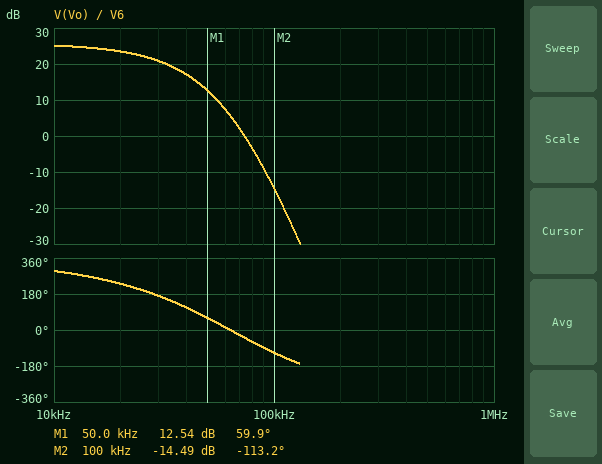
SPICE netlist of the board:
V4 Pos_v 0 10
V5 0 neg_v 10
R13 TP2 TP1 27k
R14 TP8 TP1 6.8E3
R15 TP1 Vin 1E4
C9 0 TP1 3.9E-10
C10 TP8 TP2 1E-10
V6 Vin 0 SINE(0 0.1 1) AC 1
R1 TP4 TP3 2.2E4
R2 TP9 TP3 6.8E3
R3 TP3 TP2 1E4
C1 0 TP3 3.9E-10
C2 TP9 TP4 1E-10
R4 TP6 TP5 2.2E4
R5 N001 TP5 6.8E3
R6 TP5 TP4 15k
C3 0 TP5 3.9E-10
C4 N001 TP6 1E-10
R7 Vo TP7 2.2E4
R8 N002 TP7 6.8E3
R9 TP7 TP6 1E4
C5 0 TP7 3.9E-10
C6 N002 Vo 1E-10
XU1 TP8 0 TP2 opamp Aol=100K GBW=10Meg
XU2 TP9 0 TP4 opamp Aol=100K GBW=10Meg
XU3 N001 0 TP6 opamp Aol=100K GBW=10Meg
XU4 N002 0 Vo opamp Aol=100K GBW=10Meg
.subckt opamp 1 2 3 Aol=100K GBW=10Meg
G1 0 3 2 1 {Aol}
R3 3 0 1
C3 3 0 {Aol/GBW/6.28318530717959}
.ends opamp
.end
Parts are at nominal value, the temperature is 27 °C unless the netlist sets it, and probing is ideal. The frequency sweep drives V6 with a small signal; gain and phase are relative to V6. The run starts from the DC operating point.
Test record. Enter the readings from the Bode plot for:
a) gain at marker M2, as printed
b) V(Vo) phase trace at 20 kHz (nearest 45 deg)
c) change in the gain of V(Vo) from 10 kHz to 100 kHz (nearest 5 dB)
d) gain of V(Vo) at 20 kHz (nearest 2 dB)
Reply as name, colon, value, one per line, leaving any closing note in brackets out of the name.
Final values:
gain at marker M2, as printed: -14.49 dB
V(Vo) phase trace at 20 kHz: 225 deg
change in the gain of V(Vo) from 10 kHz to 100 kHz: -40 dB
gain of V(Vo) at 20 kHz: 24 dB
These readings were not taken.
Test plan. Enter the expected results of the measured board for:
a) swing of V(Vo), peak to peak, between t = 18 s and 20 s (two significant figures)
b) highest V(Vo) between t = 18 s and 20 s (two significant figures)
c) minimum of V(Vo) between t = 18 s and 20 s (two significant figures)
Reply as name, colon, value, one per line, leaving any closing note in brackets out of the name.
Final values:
swing of V(Vo), peak to peak, between t = 18 s and 20 s: 3.8 V
highest V(Vo) between t = 18 s and 20 s: 1.9 V
minimum of V(Vo) between t = 18 s and 20 s: -1.9 V
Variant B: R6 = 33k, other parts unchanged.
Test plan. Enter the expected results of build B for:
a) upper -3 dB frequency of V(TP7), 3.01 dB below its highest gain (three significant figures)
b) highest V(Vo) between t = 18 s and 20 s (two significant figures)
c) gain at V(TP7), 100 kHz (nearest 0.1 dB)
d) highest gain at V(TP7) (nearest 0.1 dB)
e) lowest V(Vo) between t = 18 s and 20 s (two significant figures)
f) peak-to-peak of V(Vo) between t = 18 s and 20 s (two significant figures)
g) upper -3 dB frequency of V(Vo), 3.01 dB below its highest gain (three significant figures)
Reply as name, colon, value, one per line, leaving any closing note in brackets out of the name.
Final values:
upper -3 dB frequency of V(TP7), 3.01 dB below its highest gain: 49.3 kHz
highest V(Vo) between t = 18 s and 20 s: 870 mV
gain at V(TP7), 100 kHz: -27.5 dB
highest gain at V(TP7): -3.1 dB
lowest V(Vo) between t = 18 s and 20 s: -870 mV
peak-to-peak of V(Vo) between t = 18 s and 20 s: 1.7 V
upper -3 dB frequency of V(Vo), 3.01 dB below its highest gain: 25.2 kHz
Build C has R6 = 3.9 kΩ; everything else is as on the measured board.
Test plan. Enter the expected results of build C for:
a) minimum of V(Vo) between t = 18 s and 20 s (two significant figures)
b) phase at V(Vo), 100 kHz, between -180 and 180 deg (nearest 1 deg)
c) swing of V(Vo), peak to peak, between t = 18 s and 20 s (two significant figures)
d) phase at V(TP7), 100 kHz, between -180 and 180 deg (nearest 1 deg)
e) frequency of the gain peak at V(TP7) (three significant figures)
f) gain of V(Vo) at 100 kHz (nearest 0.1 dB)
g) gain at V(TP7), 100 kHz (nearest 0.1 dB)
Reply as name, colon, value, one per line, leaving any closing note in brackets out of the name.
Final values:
minimum of V(Vo) between t = 18 s and 20 s: -7.4 V
phase at V(Vo), 100 kHz, between -180 and 180 deg: -102 deg
swing of V(Vo), peak to peak, between t = 18 s and 20 s: 15 V
phase at V(TP7), 100 kHz, between -180 and 180 deg: 169 deg
frequency of the gain peak at V(TP7): 23.0 kHz
gain of V(Vo) at 100 kHz: -6.9 dB
gain at V(TP7), 100 kHz: -14.1 dB
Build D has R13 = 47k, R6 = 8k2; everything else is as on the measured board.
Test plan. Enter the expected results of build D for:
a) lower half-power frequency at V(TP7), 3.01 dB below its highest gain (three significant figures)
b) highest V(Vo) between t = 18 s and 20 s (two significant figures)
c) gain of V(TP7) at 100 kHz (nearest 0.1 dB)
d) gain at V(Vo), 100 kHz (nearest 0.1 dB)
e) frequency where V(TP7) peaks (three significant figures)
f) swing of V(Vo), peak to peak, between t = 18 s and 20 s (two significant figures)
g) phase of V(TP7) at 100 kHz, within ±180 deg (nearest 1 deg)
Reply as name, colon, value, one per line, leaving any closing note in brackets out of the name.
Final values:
lower half-power frequency at V(TP7), 3.01 dB below its highest gain: 9.90 kHz
highest V(Vo) between t = 18 s and 20 s: 6.1 V
gain of V(TP7) at 100 kHz: -18.0 dB
gain at V(Vo), 100 kHz: -10.8 dB
frequency where V(TP7) peaks: 21.8 kHz
swing of V(Vo), peak to peak, between t = 18 s and 20 s: 12 V
phase of V(TP7) at 100 kHz, within ±180 deg: 155 deg
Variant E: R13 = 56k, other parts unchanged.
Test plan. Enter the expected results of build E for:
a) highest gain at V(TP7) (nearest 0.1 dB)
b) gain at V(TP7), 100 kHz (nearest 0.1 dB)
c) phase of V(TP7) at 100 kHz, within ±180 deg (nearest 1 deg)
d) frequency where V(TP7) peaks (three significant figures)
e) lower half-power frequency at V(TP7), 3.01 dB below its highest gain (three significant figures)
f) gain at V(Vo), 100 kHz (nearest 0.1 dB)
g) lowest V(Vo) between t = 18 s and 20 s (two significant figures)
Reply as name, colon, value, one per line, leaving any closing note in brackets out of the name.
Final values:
highest gain at V(TP7): 6.1 dB
gain at V(TP7), 100 kHz: -21.9 dB
phase of V(TP7) at 100 kHz, within ±180 deg: 149 deg
frequency where V(TP7) peaks: 21.9 kHz
lower half-power frequency at V(TP7), 3.01 dB below its highest gain: 9.59 kHz
gain at V(Vo), 100 kHz: -14.7 dB
lowest V(Vo) between t = 18 s and 20 s: -4.0 V
